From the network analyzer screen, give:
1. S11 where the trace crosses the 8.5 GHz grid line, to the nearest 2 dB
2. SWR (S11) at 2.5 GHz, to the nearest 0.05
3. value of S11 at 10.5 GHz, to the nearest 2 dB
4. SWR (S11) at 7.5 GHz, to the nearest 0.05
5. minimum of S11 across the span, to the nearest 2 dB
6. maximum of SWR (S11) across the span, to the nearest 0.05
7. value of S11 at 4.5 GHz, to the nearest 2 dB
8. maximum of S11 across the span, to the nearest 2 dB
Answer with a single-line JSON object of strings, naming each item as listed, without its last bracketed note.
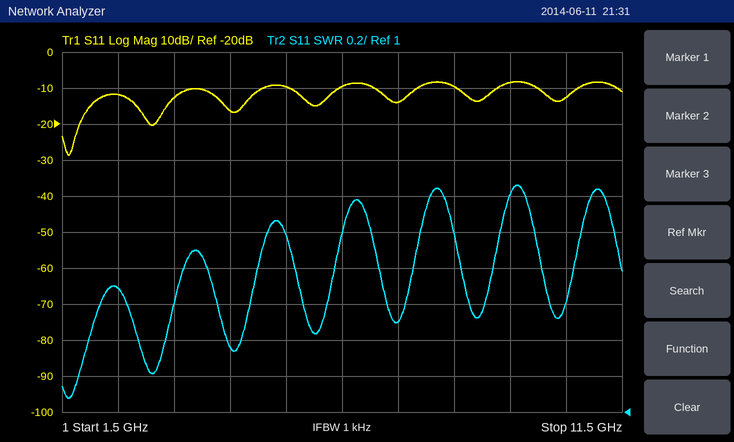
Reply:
{"S11 where the trace crosses the 8.5 GHz grid line, to the nearest 2 dB": "-10 dB", "SWR (S11) at 2.5 GHz, to the nearest 0.05": "1.70", "value of S11 at 10.5 GHz, to the nearest 2 dB": "-12 dB", "SWR (S11) at 7.5 GHz, to the nearest 0.05": "1.50", "minimum of S11 across the span, to the nearest 2 dB": "-28 dB", "maximum of SWR (S11) across the span, to the nearest 0.05": "2.25", "value of S11 at 4.5 GHz, to the nearest 2 dB": "-16 dB", "maximum of S11 across the span, to the nearest 2 dB": "-8 dB"}
